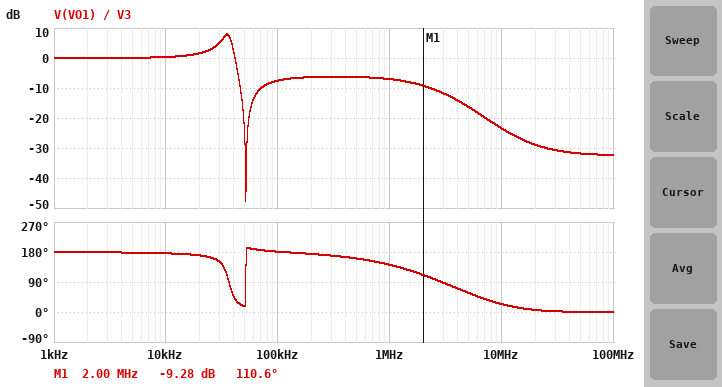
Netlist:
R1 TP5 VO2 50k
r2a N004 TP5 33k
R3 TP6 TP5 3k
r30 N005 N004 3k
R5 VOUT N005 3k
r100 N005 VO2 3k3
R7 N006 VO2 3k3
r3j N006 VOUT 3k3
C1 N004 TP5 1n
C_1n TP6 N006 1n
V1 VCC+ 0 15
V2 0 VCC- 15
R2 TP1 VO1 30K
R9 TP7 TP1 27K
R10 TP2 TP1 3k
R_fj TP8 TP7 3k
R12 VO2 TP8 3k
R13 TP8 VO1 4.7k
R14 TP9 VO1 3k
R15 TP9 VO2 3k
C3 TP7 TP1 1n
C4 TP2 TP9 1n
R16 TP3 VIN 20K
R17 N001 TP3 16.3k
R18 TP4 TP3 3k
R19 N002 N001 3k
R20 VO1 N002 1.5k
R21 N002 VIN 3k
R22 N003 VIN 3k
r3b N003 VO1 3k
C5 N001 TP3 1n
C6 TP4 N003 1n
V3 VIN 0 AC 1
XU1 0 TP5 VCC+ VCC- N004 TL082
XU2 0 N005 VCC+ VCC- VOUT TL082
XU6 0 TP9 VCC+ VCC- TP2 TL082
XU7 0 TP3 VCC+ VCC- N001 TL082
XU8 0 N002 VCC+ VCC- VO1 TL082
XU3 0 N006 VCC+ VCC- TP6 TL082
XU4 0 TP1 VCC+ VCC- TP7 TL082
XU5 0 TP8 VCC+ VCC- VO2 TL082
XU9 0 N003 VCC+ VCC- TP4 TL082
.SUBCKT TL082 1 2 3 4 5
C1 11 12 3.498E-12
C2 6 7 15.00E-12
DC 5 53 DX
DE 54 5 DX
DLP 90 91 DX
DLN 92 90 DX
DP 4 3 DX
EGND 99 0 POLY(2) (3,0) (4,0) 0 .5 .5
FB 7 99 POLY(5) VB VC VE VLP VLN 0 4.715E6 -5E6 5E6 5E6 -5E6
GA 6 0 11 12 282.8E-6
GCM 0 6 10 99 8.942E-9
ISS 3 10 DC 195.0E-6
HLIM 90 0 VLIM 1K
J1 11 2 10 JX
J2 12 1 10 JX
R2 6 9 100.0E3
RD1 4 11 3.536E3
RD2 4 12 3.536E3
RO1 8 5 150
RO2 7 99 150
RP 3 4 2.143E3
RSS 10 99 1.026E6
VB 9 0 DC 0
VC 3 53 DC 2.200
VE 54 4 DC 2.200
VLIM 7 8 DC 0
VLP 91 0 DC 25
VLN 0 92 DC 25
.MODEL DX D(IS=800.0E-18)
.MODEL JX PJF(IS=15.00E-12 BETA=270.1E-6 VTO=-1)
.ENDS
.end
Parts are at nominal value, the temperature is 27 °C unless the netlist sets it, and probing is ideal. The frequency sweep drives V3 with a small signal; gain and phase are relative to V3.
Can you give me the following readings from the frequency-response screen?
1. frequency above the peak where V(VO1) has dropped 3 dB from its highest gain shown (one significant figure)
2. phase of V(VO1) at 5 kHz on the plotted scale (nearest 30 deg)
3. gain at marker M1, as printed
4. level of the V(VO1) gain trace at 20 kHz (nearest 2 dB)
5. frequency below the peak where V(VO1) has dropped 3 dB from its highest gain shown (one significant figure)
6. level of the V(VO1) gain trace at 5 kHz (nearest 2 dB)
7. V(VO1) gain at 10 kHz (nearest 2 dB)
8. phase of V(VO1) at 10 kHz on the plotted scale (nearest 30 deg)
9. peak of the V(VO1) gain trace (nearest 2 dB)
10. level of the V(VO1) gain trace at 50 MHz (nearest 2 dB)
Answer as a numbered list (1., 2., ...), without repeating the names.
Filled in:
1. 40 kHz
2. 180 deg
3. -9.28 dB
4. 2 dB
5. 30 kHz
6. 0 dB
7. 0 dB
8. 180 deg
9. 8 dB
10. -32 dB
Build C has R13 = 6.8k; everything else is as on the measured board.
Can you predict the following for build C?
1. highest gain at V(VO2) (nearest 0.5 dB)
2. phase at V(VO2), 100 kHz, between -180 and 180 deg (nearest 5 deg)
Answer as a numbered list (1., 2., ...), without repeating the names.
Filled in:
1. 11.5 dB
2. 10 deg
